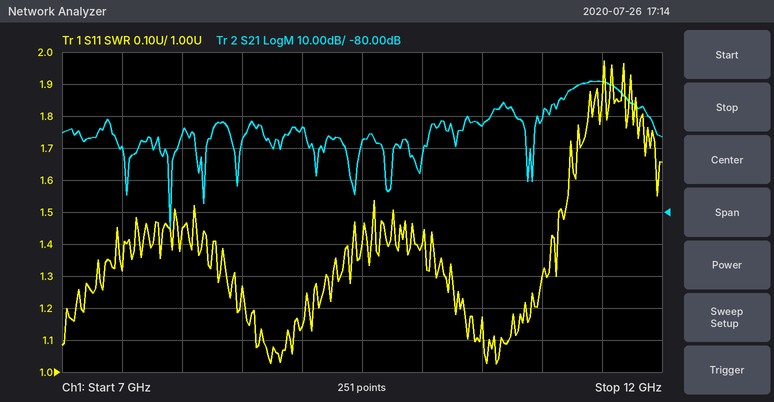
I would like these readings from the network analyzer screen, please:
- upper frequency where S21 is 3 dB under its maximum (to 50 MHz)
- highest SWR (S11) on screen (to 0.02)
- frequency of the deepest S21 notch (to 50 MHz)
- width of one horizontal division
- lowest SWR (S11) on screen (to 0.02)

11.65 GHz
1.98
7.90 GHz
500 MHz
1.02
